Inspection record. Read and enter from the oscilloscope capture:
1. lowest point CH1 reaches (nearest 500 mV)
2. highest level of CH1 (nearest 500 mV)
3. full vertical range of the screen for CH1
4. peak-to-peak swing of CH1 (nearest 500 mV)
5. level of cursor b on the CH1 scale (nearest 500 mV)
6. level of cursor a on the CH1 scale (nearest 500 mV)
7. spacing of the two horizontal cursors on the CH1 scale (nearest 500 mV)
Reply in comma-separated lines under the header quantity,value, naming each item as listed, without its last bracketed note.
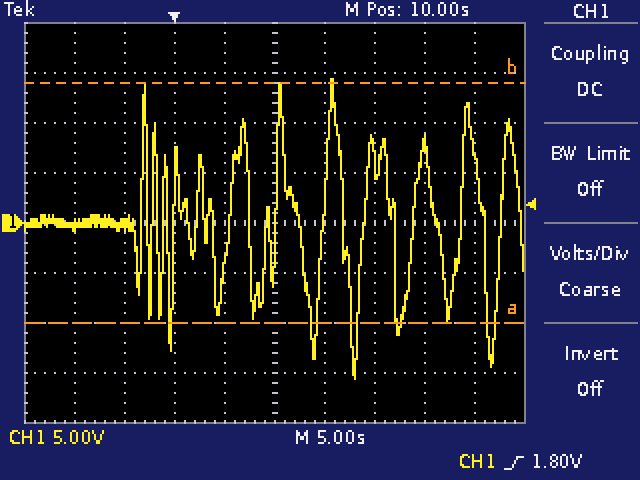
quantity,value
lowest point CH1 reaches,-15.5 V
highest level of CH1,14.5 V
full vertical range of the screen for CH1,40 V
peak-to-peak swing of CH1,30.0 V
level of cursor b on the CH1 scale,14.0 V
level of cursor a on the CH1 scale,-10.0 V
spacing of the two horizontal cursors on the CH1 scale,24.0 V
